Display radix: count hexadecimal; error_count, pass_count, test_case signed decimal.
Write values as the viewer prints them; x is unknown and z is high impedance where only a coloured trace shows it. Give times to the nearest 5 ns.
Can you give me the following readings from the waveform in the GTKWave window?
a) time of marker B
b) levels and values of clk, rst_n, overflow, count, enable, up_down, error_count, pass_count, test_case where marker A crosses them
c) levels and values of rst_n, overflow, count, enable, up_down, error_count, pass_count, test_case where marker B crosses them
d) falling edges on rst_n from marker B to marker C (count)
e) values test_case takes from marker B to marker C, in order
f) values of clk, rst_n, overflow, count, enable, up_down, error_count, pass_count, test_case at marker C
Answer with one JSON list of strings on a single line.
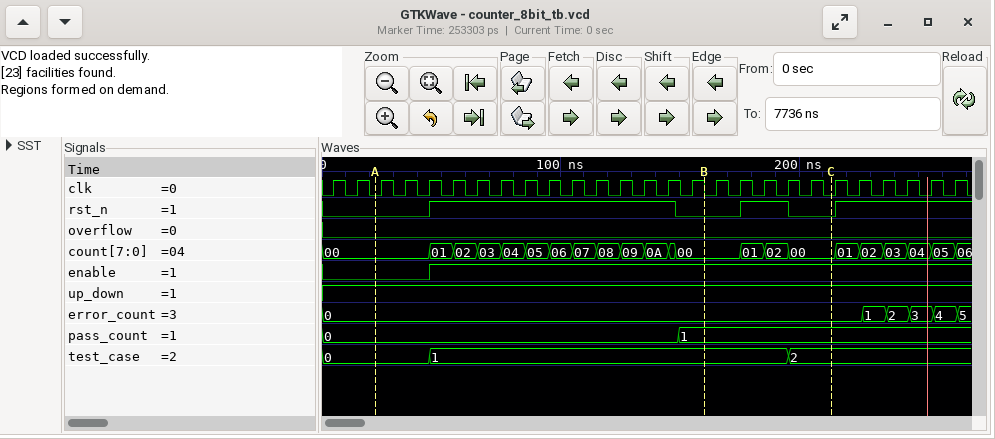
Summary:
["160 ns", "clk=0, rst_n=0, overflow=0, count=00, enable=0, up_down=1, error_count=0, pass_count=0, test_case=0", "rst_n=0, overflow=0, count=00, enable=1, up_down=1, error_count=0, pass_count=1, test_case=1", "1", "1, 2", "clk=0, rst_n=0, overflow=0, count=00, enable=1, up_down=1, error_count=0, pass_count=1, test_case=2"]
